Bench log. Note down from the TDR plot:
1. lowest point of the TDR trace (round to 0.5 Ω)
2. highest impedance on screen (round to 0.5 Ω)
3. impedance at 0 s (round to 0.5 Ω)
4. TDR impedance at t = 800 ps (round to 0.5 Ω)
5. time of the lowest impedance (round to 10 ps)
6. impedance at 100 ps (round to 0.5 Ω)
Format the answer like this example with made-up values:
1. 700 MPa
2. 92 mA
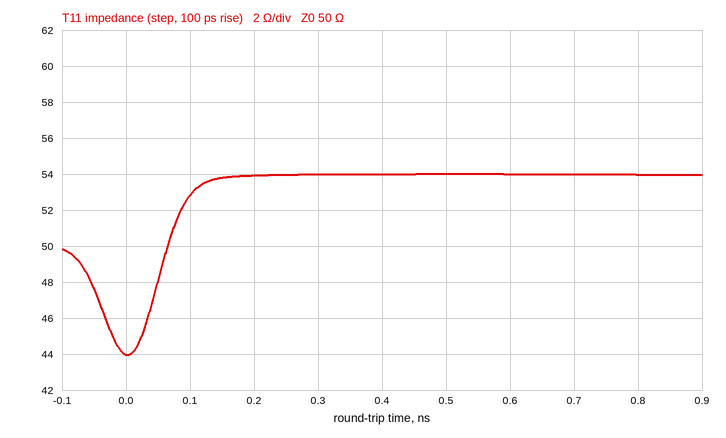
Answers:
1. 44.0 Ω
2. 54.0 Ω
3. 44.0 Ω
4. 54.0 Ω
5. 0 ps
6. 53.0 Ω
